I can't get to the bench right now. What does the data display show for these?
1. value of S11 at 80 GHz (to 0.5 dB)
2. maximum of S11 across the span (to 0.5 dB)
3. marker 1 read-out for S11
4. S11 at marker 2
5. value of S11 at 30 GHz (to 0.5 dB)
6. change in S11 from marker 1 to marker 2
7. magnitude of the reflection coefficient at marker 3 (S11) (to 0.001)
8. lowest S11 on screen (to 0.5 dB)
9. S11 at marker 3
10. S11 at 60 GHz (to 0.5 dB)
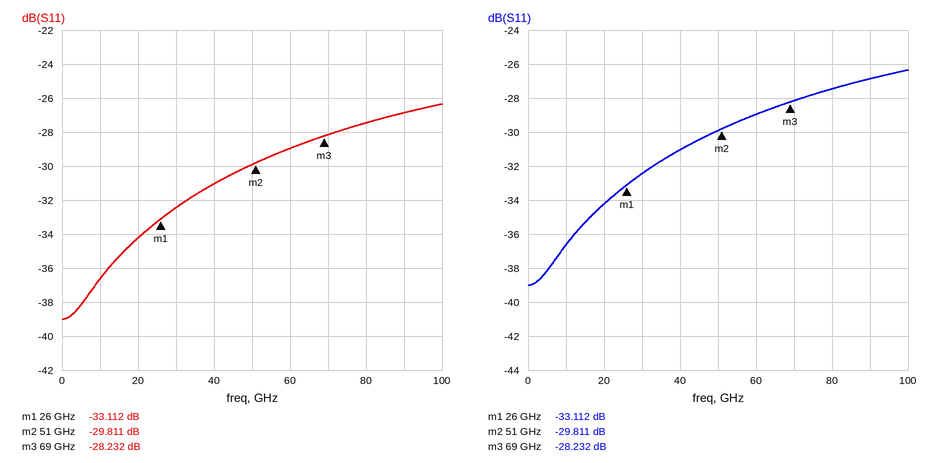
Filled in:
-27.5 dB
-26.5 dB
-33.112 dB
-29.811 dB
-32.5 dB
3.301 dB
0.039
-39.0 dB
-28.232 dB
-29.0 dB
